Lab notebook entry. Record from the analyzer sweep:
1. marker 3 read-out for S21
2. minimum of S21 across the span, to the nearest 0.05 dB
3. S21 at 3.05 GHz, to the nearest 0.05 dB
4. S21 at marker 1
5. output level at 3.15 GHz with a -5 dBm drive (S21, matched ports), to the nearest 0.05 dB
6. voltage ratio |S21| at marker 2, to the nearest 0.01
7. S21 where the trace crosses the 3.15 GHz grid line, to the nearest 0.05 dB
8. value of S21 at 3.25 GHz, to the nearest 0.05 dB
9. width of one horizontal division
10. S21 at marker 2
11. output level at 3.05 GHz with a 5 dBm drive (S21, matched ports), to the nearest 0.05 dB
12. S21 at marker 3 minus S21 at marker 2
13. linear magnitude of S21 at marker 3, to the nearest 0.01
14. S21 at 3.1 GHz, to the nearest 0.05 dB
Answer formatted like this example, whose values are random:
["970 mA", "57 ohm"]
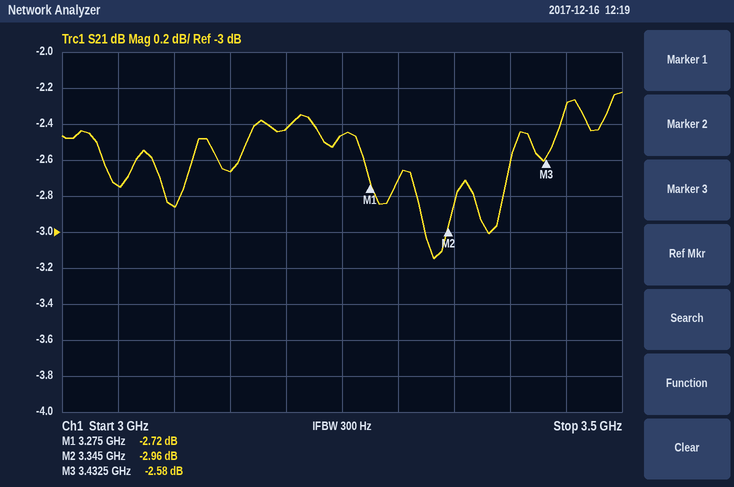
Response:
["-2.58 dB", "-3.15 dB", "-2.75 dB", "-2.72 dB", "-7.65 dBm", "0.71", "-2.65 dB", "-2.45 dB", "50 MHz", "-2.96 dB", "2.25 dBm", "0.38 dB", "0.74", "-2.85 dB"]
